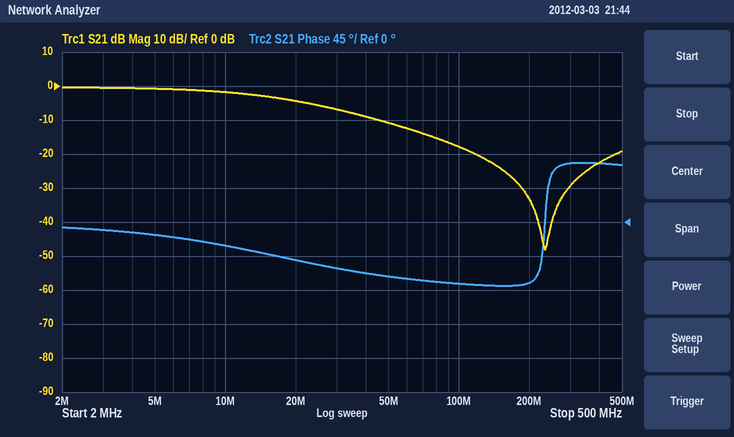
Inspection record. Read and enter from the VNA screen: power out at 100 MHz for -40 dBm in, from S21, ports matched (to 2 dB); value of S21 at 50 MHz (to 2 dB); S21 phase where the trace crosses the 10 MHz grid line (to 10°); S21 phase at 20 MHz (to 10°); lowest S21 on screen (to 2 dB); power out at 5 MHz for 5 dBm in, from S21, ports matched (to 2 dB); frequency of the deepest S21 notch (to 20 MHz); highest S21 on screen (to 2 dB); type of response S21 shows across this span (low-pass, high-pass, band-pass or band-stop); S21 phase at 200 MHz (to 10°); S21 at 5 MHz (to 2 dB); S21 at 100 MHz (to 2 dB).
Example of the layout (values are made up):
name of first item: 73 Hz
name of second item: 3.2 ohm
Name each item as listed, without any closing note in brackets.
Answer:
power out at 100 MHz for -40 dBm in, from S21, ports matched: -58 dBm
value of S21 at 50 MHz: -10 dB
S21 phase where the trace crosses the 10 MHz grid line: -30°
S21 phase at 20 MHz: -50°
lowest S21 on screen: -48 dB
power out at 5 MHz for 5 dBm in, from S21, ports matched: 4 dBm
frequency of the deepest S21 notch: 240 MHz
highest S21 on screen: 0 dB
type of response S21 shows across this span: low-pass
S21 phase at 200 MHz: -80°
S21 at 5 MHz: 0 dB
S21 at 100 MHz: -18 dB
